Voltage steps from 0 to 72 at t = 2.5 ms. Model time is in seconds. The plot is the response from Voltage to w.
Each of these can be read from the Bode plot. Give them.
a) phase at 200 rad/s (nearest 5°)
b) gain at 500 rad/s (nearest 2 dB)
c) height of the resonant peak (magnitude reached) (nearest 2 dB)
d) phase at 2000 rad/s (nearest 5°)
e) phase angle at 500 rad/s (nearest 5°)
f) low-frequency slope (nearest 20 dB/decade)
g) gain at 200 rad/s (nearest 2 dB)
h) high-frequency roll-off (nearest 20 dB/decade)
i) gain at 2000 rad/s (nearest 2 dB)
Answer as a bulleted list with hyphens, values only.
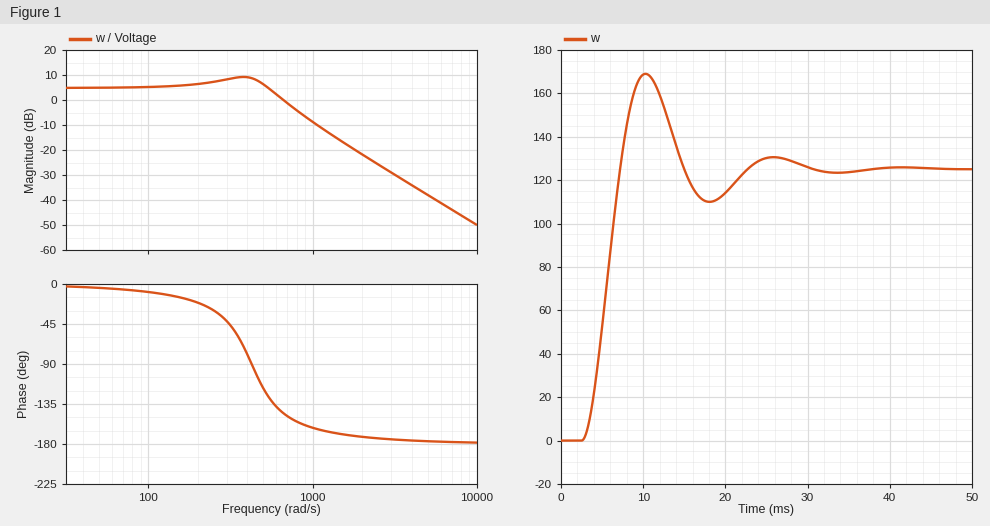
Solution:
- -20°
- 6 dB
- 10 dB
- -170°
- -115°
- 0 dB/decade
- 6 dB
- -40 dB/decade
- -22 dB
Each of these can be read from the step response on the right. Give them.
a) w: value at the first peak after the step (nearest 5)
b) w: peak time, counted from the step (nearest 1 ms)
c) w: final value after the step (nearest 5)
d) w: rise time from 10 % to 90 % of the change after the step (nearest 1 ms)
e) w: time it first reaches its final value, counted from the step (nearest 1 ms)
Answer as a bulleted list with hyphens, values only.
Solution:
- 170
- 8 ms
- 125
- 3 ms
- 5 ms
